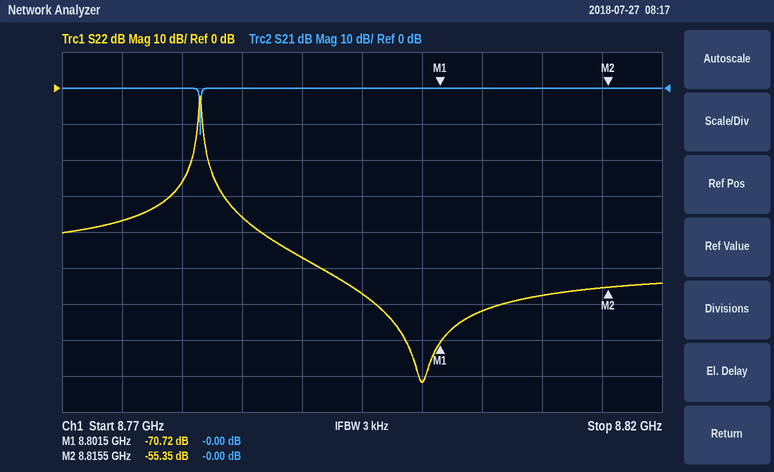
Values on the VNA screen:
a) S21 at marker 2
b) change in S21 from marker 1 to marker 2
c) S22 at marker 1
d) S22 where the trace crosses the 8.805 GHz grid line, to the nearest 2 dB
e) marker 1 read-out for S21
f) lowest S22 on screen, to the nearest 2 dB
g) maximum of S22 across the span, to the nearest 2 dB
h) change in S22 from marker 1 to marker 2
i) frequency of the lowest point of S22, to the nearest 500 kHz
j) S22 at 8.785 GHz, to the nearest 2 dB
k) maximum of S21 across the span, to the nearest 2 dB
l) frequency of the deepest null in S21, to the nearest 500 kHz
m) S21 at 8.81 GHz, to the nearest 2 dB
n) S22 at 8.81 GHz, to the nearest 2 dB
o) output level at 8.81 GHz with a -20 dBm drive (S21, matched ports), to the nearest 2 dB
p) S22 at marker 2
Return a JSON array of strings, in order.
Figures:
["-0.00 dB", "0.00 dB", "-70.72 dB", "-62 dB", "-0.00 dB", "-82 dB", "-2 dB", "15.37 dB", "8.8000 GHz", "-36 dB", "0 dB", "8.7815 GHz", "0 dB", "-58 dB", "-20 dBm", "-55.35 dB"]
